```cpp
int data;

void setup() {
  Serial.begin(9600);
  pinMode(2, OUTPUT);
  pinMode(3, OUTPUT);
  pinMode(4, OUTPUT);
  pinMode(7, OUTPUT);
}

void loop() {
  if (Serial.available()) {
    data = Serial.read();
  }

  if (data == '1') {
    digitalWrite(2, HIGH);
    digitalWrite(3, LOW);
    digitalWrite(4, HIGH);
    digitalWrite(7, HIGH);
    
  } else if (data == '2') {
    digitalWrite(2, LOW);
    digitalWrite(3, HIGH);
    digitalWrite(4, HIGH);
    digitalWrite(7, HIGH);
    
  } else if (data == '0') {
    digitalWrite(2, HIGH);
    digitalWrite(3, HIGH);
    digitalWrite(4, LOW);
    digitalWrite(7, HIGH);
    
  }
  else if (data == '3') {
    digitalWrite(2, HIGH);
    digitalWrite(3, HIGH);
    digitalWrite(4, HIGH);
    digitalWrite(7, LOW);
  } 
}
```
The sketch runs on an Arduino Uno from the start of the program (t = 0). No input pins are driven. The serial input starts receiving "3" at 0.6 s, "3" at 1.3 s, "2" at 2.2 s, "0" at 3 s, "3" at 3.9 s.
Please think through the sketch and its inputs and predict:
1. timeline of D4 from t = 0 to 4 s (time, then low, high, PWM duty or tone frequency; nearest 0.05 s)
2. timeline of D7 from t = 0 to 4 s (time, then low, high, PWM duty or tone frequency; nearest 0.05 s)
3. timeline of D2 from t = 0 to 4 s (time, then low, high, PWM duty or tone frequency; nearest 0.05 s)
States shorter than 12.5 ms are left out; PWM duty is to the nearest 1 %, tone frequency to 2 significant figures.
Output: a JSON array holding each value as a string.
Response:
["0 s low; 0.6 s high; 3 s low; 3.9 s high", "0 s low; 2.2 s high; 3.9 s low", "0 s low; 0.6 s high; 2.2 s low; 3 s high"]
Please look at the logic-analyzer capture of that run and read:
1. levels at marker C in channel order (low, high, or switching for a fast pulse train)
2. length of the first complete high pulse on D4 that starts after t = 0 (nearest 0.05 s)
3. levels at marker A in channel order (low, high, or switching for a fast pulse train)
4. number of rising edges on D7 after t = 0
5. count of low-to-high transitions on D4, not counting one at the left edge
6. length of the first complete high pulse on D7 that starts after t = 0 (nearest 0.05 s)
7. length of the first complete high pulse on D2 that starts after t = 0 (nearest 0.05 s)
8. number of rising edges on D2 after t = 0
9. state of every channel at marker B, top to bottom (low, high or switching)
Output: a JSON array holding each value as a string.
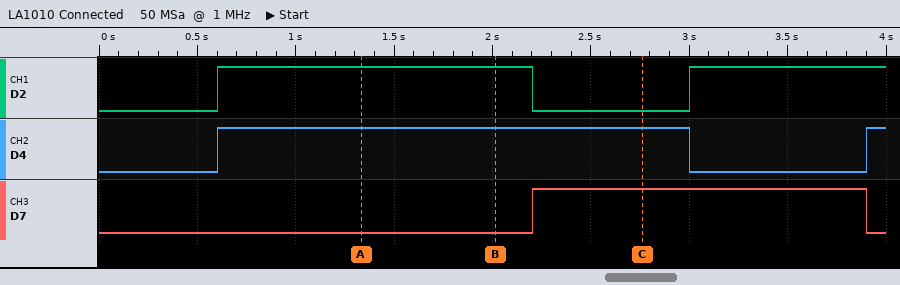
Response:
["D2 low, D4 high, D7 high", "2.40 s", "D2 high, D4 high, D7 low", "1", "2", "1.70 s", "1.60 s", "2", "D2 high, D4 high, D7 low"]
